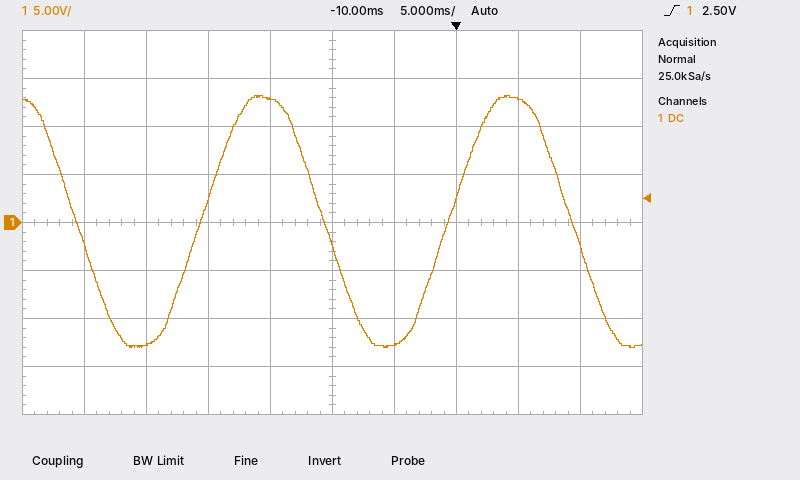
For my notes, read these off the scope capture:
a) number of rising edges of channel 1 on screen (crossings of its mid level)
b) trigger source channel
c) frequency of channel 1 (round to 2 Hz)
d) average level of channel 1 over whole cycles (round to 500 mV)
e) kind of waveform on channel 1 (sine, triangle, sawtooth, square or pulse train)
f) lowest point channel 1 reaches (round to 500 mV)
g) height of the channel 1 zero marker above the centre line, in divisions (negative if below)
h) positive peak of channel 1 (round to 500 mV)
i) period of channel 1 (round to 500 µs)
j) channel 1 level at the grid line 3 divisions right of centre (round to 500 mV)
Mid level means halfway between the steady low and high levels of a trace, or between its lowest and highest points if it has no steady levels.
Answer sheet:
2
channel 1
50 Hz
0.0 V
sine
-13.0 V
0.0 div
13.0 V
20.0 ms
13.0 V
